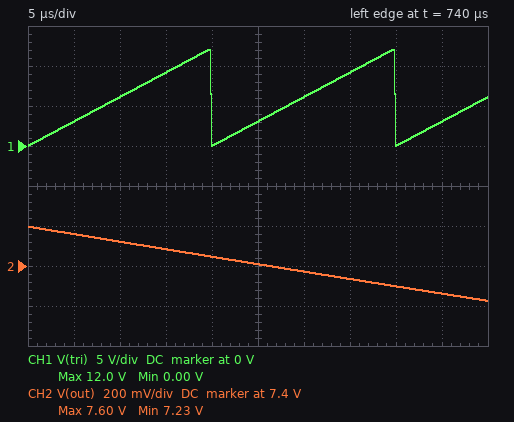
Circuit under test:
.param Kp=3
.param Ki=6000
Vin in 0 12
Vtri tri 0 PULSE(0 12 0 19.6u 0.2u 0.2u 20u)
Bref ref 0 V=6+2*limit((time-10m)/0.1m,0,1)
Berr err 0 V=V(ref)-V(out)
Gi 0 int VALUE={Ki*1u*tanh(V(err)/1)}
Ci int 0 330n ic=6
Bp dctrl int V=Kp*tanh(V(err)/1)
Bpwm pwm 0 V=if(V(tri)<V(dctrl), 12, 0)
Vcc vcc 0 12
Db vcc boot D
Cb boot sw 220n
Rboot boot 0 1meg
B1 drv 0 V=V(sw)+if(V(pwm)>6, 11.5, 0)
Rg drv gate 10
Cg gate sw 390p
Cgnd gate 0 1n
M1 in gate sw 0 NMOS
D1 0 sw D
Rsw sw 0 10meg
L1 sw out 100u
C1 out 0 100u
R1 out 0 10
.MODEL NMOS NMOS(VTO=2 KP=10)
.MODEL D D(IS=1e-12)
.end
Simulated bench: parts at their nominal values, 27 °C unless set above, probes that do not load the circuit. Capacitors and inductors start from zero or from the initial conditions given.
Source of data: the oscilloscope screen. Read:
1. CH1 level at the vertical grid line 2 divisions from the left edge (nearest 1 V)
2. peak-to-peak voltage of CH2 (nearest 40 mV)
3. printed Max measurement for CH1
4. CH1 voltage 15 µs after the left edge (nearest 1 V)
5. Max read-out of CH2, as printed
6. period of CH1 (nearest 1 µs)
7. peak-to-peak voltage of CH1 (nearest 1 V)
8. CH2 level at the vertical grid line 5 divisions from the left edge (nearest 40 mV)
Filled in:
6 V
360 mV
12.0 V
9 V
7.60 V
20 µs
12 V
7.40 V
